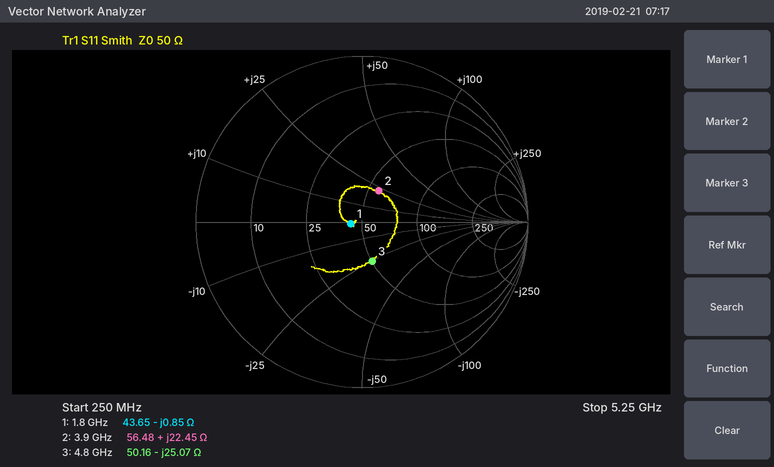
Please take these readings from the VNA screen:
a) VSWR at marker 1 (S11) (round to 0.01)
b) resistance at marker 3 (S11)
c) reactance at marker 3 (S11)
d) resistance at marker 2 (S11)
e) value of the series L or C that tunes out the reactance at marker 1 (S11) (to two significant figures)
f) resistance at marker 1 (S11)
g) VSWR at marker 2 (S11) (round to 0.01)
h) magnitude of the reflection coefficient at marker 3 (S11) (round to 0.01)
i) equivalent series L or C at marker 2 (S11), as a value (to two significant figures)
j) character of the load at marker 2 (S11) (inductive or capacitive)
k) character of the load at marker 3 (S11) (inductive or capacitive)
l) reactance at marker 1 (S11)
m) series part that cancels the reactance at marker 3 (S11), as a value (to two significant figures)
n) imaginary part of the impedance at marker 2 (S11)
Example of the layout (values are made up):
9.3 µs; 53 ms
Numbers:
1.15; 50.16 Ω; -25.07 Ω; 56.48 Ω; 75 pH; 43.65 Ω; 1.55; 0.24; 920 pH; inductive; capacitive; -0.85 Ω; 830 pH; +22.45 Ω
